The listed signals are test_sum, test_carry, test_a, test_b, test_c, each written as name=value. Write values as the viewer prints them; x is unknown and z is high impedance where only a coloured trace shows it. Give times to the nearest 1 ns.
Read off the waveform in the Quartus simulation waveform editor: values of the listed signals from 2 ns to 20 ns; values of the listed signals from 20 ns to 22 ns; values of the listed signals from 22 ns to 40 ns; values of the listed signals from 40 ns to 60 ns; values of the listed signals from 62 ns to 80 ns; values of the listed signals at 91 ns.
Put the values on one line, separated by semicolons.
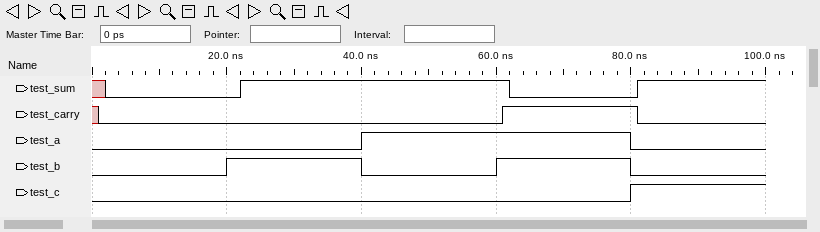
test_sum=0, test_carry=0, test_a=0, test_b=0, test_c=0; test_sum=0, test_carry=0, test_a=0, test_b=1, test_c=0; test_sum=1, test_carry=0, test_a=0, test_b=1, test_c=0; test_sum=1, test_carry=0, test_a=1, test_b=0, test_c=0; test_sum=0, test_carry=1, test_a=1, test_b=1, test_c=0; test_sum=1, test_carry=0, test_a=0, test_b=0, test_c=1
